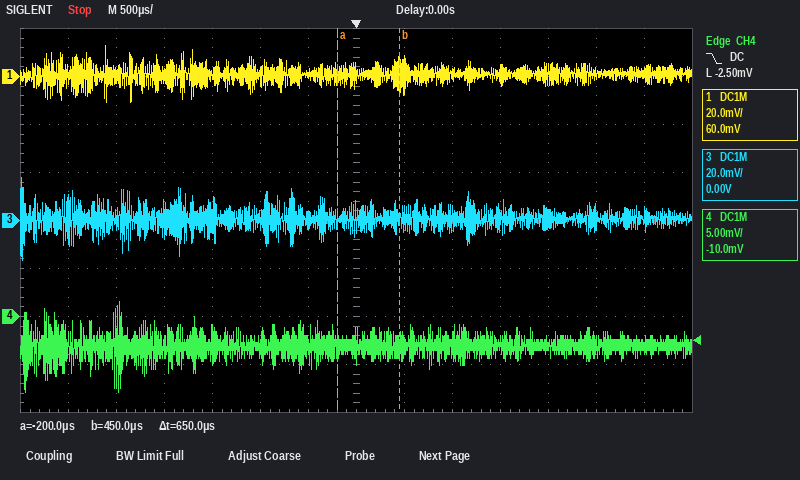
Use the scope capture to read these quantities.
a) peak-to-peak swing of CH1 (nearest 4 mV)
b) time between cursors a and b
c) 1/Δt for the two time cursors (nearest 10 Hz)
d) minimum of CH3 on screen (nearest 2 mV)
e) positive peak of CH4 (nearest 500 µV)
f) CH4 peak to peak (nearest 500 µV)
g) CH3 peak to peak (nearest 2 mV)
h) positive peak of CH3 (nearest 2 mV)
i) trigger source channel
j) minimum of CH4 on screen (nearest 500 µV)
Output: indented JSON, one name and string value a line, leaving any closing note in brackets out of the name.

{
  "peak-to-peak swing of CH1": "24 mV",
  "time between cursors a and b": "650 µs",
  "1/Δt for the two time cursors": "1.54 kHz",
  "minimum of CH3 on screen": "-16 mV",
  "positive peak of CH4": "1.5 mV",
  "CH4 peak to peak": "9.5 mV",
  "CH3 peak to peak": "34 mV",
  "positive peak of CH3": "18 mV",
  "trigger source channel": "CH4",
  "minimum of CH4 on screen": "-8.0 mV"
}
